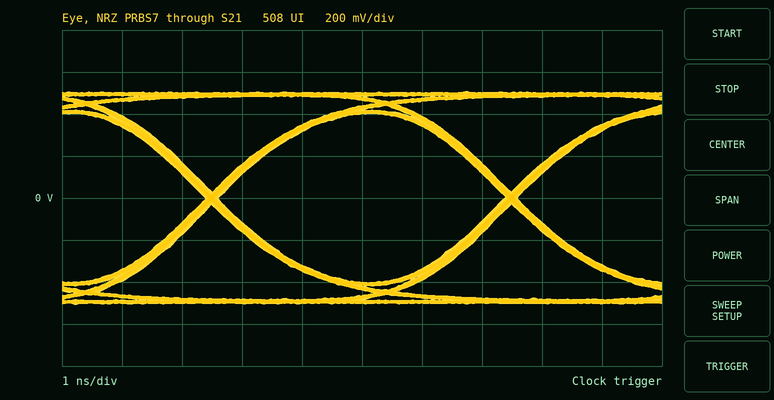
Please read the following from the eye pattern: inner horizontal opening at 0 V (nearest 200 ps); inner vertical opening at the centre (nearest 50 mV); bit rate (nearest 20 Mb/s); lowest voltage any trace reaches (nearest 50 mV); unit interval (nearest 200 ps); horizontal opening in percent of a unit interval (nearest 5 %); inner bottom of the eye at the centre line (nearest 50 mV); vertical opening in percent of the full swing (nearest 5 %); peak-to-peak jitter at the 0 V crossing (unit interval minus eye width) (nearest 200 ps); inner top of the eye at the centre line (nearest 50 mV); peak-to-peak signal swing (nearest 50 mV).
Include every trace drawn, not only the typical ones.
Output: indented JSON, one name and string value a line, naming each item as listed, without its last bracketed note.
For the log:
{
  "inner horizontal opening at 0 V": "4.8 ns",
  "inner vertical opening at the centre": "800 mV",
  "bit rate": "200 Mb/s",
  "lowest voltage any trace reaches": "-500 mV",
  "unit interval": "5.0 ns",
  "horizontal opening in percent of a unit interval": "95 %",
  "inner bottom of the eye at the centre line": "-400 mV",
  "vertical opening in percent of the full swing": "80 %",
  "peak-to-peak jitter at the 0 V crossing (unit interval minus eye width)": "200 ps",
  "inner top of the eye at the centre line": "400 mV",
  "peak-to-peak signal swing": "1.00 V"
}
